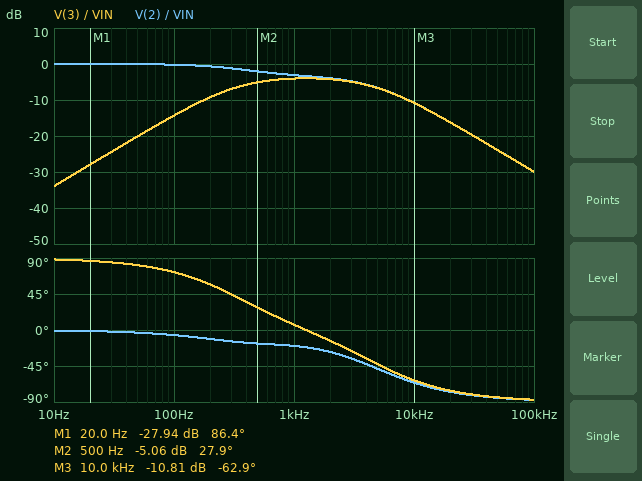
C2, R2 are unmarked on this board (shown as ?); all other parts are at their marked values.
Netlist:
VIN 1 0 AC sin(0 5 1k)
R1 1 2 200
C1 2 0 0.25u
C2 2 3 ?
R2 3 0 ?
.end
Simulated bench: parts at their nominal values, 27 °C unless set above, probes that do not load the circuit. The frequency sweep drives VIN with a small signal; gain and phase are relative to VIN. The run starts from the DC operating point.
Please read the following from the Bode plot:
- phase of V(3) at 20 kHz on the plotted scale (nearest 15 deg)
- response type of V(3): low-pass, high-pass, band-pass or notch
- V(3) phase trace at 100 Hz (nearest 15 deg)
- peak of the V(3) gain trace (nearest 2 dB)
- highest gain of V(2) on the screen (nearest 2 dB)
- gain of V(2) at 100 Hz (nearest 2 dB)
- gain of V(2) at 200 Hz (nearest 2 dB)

-75 deg
band-pass
75 deg
-4 dB
0 dB
0 dB
0 dB
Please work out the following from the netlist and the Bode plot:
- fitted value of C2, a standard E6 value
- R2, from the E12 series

680 nF
470 Ω
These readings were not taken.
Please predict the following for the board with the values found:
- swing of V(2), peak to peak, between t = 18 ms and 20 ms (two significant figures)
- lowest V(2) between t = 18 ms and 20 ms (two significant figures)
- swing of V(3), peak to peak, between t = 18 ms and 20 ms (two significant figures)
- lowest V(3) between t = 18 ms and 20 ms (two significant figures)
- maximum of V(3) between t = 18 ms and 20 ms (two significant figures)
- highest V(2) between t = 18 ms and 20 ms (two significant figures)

7.0 V
-3.5 V
6.3 V
-3.1 V
3.1 V
3.5 V
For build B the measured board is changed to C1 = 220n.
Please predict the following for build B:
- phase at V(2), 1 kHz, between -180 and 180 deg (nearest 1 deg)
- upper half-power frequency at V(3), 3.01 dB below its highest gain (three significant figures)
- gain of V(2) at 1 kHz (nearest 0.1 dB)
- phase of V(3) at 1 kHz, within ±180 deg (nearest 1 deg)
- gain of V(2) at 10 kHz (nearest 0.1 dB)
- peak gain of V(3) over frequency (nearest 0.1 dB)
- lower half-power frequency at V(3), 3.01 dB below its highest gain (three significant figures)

-18 deg
5.96 kHz
-3.0 dB
8 deg
-9.9 dB
-3.9 dB
302 Hz
